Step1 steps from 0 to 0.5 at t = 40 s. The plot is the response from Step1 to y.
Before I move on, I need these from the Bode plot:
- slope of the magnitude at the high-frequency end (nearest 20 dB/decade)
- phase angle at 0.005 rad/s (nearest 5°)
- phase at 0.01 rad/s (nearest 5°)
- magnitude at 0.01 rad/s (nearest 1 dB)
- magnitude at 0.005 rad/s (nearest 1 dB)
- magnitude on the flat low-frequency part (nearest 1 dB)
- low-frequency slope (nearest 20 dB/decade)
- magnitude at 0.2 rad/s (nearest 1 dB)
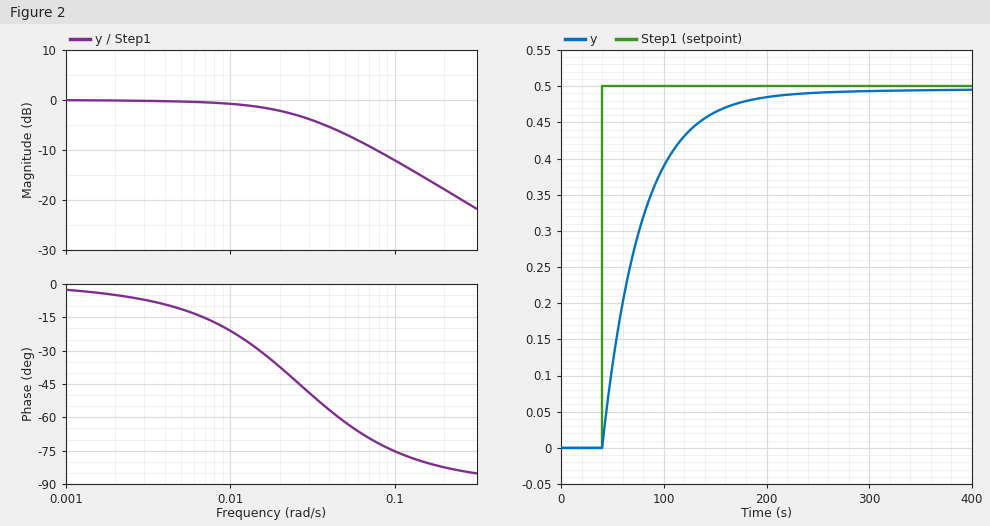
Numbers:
-20 dB/decade
-10°
-20°
-1 dB
0 dB
0 dB
0 dB/decade
-18 dB
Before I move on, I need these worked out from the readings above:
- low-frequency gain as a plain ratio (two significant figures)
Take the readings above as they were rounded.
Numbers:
1.0
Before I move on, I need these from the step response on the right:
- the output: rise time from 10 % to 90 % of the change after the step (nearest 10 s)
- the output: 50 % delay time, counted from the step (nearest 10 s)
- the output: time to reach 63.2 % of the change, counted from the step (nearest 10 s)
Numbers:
90 s
30 s
40 s
